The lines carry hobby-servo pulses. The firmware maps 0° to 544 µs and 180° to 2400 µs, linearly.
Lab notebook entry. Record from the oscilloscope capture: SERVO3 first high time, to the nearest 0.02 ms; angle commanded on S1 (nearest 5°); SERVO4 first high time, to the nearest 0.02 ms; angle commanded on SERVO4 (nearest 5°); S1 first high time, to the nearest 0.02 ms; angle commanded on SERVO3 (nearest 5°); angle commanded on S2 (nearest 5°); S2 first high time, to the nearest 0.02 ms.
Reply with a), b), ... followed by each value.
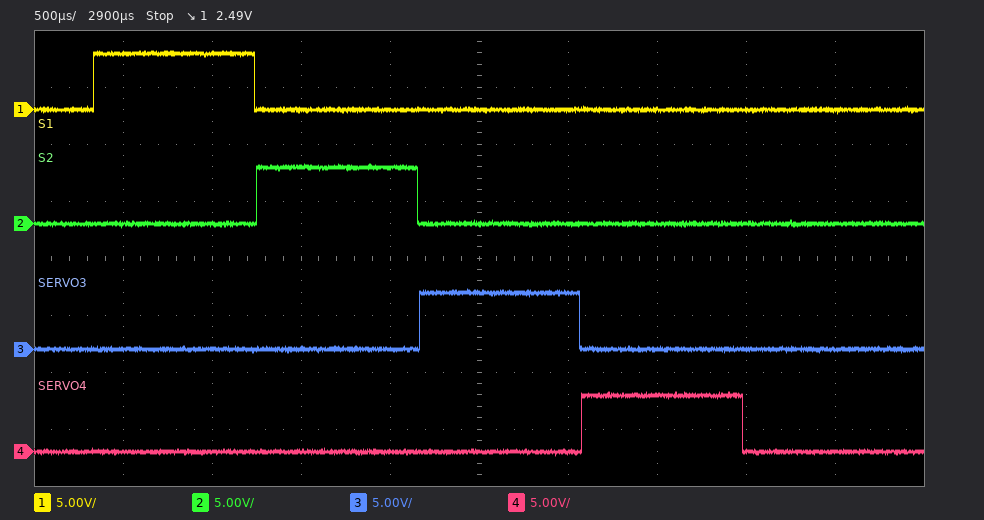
a) 0.90 ms
b) 35°
c) 0.90 ms
d) 35°
e) 0.90 ms
f) 35°
g) 35°
h) 0.90 ms
